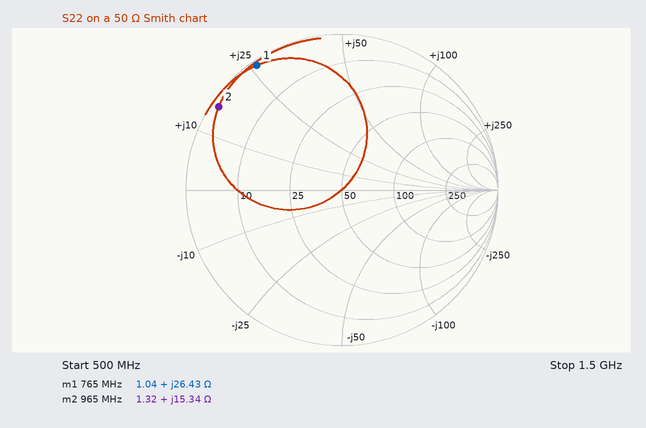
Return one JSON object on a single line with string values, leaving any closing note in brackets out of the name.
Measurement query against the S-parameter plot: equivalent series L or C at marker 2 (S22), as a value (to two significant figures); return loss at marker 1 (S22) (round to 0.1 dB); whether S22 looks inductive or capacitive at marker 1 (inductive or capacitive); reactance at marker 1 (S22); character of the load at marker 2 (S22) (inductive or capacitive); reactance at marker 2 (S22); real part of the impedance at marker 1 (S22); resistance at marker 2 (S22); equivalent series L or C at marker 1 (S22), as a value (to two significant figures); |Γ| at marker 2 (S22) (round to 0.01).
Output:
{"equivalent series L or C at marker 2 (S22), as a value": "2.5 nH", "return loss at marker 1 (S22)": "0.3 dB", "whether S22 looks inductive or capacitive at marker 1": "inductive", "reactance at marker 1": "+26.43 Ω", "character of the load at marker 2 (S22)": "inductive", "reactance at marker 2": "+15.34 Ω", "real part of the impedance at marker 1": "1.04 Ω", "resistance at marker 2": "1.32 Ω", "equivalent series L or C at marker 1 (S22), as a value": "5.5 nH", "|Γ| at marker 2 (S22)": "0.95"}
